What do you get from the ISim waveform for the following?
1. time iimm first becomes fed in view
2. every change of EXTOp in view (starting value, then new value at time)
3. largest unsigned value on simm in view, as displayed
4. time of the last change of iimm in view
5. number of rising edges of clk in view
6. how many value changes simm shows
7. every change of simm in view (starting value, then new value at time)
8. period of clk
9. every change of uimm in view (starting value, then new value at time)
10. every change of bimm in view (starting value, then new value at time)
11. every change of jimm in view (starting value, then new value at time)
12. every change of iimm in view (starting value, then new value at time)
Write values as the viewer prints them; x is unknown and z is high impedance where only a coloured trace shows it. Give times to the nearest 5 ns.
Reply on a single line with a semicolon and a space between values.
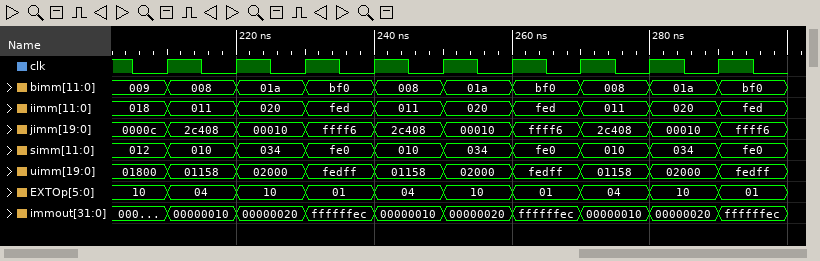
230 ns; 10, 04 at 210 ns, 10 at 220 ns, 01 at 230 ns, 04 at 240 ns, 10 at 250 ns, 01 at 260 ns, 04 at 270 ns, 10 at 280 ns, 01 at 290 ns; fe0; 290 ns; 9; 9; 012, 010 at 210 ns, 034 at 220 ns, fe0 at 230 ns, 010 at 240 ns, 034 at 250 ns, fe0 at 260 ns, 010 at 270 ns, 034 at 280 ns, fe0 at 290 ns; 10 ns; 01800, 01158 at 210 ns, 02000 at 220 ns, fedff at 230 ns, 01158 at 240 ns, 02000 at 250 ns, fedff at 260 ns, 01158 at 270 ns, 02000 at 280 ns, fedff at 290 ns; 009, 008 at 210 ns, 01a at 220 ns, bf0 at 230 ns, 008 at 240 ns, 01a at 250 ns, bf0 at 260 ns, 008 at 270 ns, 01a at 280 ns, bf0 at 290 ns; 0000c, 2c408 at 210 ns, 00010 at 220 ns, ffff6 at 230 ns, 2c408 at 240 ns, 00010 at 250 ns, ffff6 at 260 ns, 2c408 at 270 ns, 00010 at 280 ns, ffff6 at 290 ns; 018, 011 at 210 ns, 020 at 220 ns, fed at 230 ns, 011 at 240 ns, 020 at 250 ns, fed at 260 ns, 011 at 270 ns, 020 at 280 ns, fed at 290 ns
